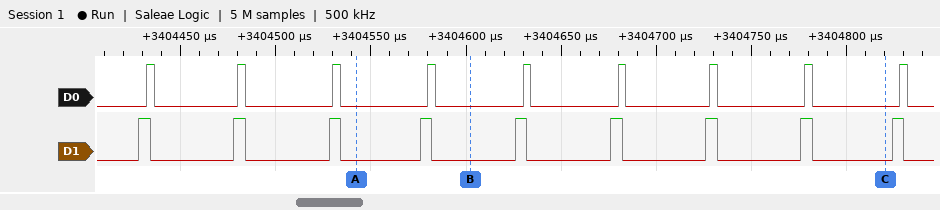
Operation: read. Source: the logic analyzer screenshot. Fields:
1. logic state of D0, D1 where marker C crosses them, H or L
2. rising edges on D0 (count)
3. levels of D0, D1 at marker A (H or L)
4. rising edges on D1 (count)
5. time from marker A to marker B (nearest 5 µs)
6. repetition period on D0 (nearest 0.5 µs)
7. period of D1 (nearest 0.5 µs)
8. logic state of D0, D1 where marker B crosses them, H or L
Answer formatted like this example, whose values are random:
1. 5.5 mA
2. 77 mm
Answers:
1. D0=L, D1=L
2. 9
3. D0=L, D1=L
4. 9
5. 60 µs
6. 49.5 µs
7. 49.5 µs
8. D0=L, D1=L
